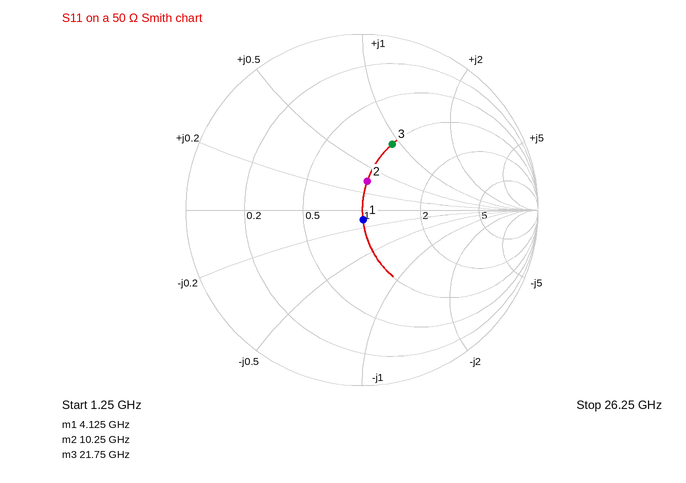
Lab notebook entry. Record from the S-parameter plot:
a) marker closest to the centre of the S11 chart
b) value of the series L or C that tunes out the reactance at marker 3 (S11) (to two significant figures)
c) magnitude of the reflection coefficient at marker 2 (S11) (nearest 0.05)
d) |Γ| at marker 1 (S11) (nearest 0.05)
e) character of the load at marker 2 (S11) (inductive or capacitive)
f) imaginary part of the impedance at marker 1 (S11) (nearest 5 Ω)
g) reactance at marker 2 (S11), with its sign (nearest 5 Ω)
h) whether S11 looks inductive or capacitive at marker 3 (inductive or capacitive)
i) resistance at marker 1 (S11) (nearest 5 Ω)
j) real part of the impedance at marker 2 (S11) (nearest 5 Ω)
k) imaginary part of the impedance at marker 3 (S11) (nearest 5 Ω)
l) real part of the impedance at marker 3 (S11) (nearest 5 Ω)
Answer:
marker 1
160 fF
0.15
0.05
inductive
-5 Ω
+15 Ω
inductive
50 Ω
50 Ω
+45 Ω
50 Ω
